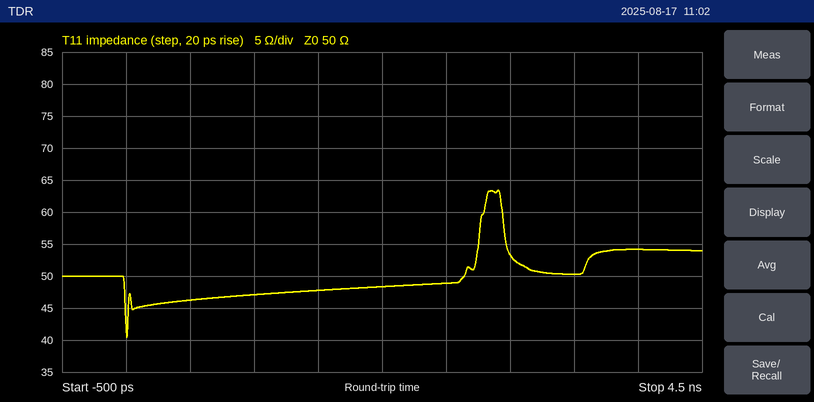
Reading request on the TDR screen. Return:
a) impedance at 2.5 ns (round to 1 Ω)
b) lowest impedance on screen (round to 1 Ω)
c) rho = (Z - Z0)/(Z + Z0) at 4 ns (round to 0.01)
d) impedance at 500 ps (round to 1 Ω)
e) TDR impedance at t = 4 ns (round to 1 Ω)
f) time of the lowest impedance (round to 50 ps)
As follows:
49 Ω
40 Ω
+0.04
46 Ω
54 Ω
0 ps
